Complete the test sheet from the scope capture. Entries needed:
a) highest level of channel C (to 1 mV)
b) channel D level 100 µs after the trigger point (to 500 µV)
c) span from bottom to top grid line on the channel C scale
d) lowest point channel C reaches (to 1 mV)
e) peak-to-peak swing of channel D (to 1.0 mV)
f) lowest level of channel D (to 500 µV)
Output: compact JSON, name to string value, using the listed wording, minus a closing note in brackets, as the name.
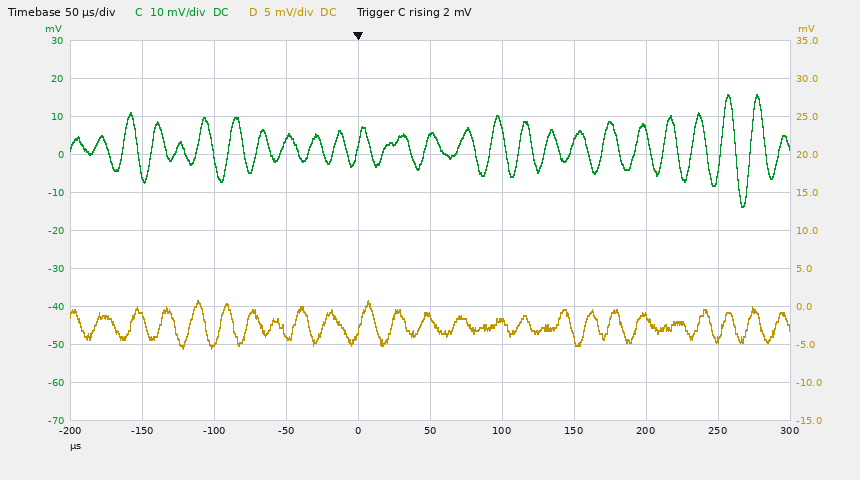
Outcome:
{"highest level of channel C": "16 mV", "channel D level 100 µs after the trigger point": "-2.0 mV", "span from bottom to top grid line on the channel C scale": "100 mV", "lowest point channel C reaches": "-14 mV", "peak-to-peak swing of channel D": "6.0 mV", "lowest level of channel D": "-5.5 mV"}
